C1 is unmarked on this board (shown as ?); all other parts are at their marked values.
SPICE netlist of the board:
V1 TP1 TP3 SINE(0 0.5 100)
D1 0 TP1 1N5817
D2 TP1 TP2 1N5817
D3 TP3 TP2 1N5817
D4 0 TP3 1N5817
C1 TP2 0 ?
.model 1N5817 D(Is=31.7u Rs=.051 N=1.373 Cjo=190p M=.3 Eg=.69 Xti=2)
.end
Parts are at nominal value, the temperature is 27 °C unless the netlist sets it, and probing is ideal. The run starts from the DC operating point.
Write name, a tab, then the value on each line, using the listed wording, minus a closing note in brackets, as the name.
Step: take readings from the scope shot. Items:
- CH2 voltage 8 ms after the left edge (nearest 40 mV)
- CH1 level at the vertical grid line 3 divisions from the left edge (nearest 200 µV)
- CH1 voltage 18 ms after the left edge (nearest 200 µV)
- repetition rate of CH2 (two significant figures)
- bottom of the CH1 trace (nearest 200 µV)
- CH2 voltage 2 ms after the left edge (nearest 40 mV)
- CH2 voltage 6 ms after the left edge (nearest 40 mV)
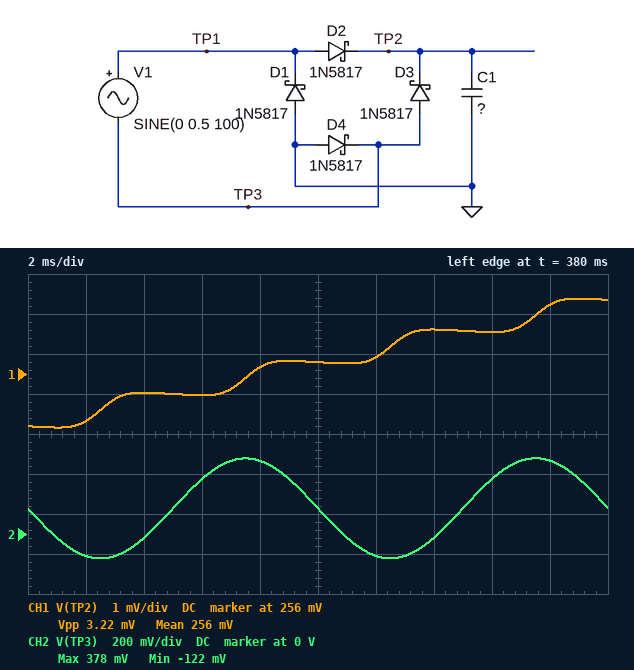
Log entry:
CH2 voltage 8 ms after the left edge	360 mV
CH1 level at the vertical grid line 3 divisions from the left edge	255.4 mV
CH1 voltage 18 ms after the left edge	257.8 mV
repetition rate of CH2	100 Hz
bottom of the CH1 trace	254.6 mV
CH2 voltage 2 ms after the left edge	-120 mV
CH2 voltage 6 ms after the left edge	280 mV
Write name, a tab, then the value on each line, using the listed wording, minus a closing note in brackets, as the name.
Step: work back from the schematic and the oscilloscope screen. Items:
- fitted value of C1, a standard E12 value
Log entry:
fitted value of C1, a standard E12 value	1.5 mF
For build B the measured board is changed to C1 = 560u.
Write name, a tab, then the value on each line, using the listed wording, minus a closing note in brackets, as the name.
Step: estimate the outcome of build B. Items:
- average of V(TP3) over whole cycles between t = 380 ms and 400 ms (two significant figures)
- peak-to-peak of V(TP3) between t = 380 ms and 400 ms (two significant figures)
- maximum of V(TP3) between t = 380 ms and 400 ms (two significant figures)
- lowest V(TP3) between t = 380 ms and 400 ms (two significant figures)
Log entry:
average of V(TP3) over whole cycles between t = 380 ms and 400 ms	160 mV
peak-to-peak of V(TP3) between t = 380 ms and 400 ms	500 mV
maximum of V(TP3) between t = 380 ms and 400 ms	410 mV
lowest V(TP3) between t = 380 ms and 400 ms	-94 mV
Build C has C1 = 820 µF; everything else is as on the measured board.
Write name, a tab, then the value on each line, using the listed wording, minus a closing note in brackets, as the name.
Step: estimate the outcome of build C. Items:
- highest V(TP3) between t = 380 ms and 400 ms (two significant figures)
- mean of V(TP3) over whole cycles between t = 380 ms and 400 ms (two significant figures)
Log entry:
highest V(TP3) between t = 380 ms and 400 ms	400 mV
mean of V(TP3) over whole cycles between t = 380 ms and 400 ms	150 mV
